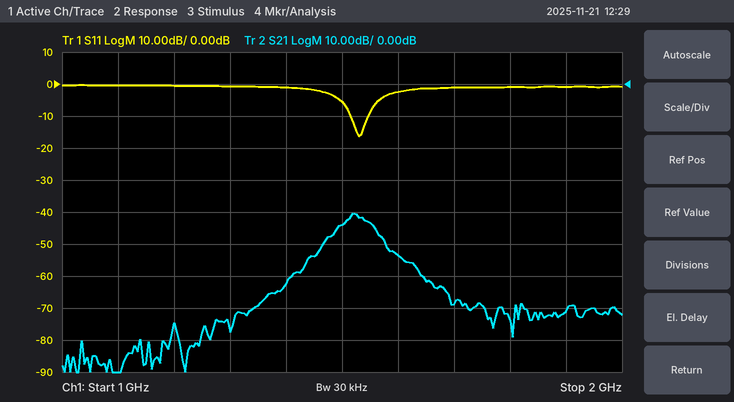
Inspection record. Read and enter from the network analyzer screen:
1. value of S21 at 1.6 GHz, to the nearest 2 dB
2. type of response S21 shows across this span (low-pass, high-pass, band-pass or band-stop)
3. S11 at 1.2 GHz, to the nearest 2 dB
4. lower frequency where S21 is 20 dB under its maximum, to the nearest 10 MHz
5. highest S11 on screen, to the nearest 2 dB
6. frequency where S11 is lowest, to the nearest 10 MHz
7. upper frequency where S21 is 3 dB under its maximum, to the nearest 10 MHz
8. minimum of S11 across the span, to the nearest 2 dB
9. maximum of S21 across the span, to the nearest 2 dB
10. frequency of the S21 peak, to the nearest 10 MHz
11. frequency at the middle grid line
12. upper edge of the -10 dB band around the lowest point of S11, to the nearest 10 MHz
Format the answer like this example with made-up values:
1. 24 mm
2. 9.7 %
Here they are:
1. -54 dB
2. band-pass
3. 0 dB
4. 1.41 GHz
5. 0 dB
6. 1.53 GHz
7. 1.55 GHz
8. -16 dB
9. -40 dB
10. 1.52 GHz
11. 1.5 GHz
12. 1.55 GHz
